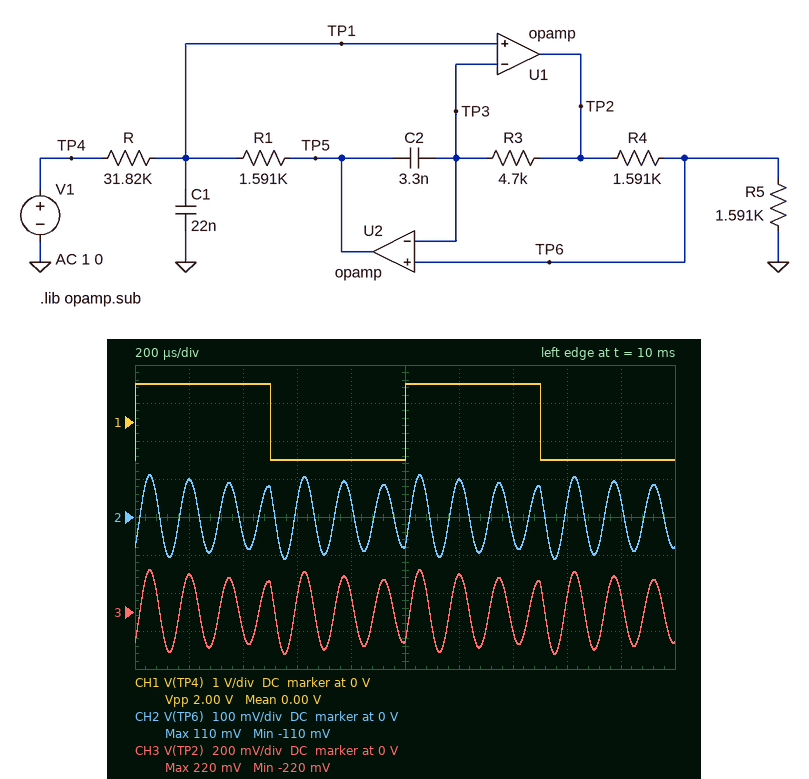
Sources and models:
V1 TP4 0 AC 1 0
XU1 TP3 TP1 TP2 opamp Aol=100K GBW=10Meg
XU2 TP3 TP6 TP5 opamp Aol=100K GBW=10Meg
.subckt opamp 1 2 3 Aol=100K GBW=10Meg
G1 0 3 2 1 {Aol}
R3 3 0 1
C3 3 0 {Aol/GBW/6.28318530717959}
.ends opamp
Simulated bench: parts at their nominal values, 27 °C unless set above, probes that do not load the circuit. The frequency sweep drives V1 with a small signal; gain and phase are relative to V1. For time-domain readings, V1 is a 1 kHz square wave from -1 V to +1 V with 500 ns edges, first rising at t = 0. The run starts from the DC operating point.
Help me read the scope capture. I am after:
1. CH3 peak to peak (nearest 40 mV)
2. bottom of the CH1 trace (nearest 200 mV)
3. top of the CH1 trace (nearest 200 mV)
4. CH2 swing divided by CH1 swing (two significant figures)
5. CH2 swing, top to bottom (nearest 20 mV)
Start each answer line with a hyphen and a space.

- 440 mV
- -1.0 V
- 1.0 V
- 0.11
- 220 mV
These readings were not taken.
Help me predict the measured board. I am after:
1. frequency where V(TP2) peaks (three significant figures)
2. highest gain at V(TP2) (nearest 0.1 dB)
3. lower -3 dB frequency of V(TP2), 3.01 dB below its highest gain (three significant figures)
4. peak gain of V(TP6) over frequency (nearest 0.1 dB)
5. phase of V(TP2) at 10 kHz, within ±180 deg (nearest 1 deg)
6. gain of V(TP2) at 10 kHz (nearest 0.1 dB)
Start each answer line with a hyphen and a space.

- 6.82 kHz
- 6.0 dB
- 6.71 kHz
- 0 dB
- -88 deg
- -21.4 dB
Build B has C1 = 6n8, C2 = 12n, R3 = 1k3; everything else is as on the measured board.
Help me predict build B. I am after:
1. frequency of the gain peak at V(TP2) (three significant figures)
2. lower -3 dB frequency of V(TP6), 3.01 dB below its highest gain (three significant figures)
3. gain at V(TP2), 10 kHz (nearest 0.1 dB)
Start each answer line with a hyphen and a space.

- 12.2 kHz
- 11.9 kHz
- -10.6 dB
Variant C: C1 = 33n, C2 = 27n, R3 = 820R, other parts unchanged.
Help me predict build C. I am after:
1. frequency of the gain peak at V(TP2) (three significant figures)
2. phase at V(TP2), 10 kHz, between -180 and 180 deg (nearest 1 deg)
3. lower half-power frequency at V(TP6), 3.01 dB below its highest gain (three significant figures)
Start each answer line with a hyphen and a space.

- 4.66 kHz
- -89 deg
- 4.59 kHz
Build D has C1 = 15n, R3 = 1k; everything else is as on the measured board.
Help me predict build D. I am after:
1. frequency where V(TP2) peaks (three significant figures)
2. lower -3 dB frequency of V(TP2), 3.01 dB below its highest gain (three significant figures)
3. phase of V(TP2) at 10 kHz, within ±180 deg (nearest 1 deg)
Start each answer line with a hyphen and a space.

- 17.8 kHz
- 17.7 kHz
- 89 deg
